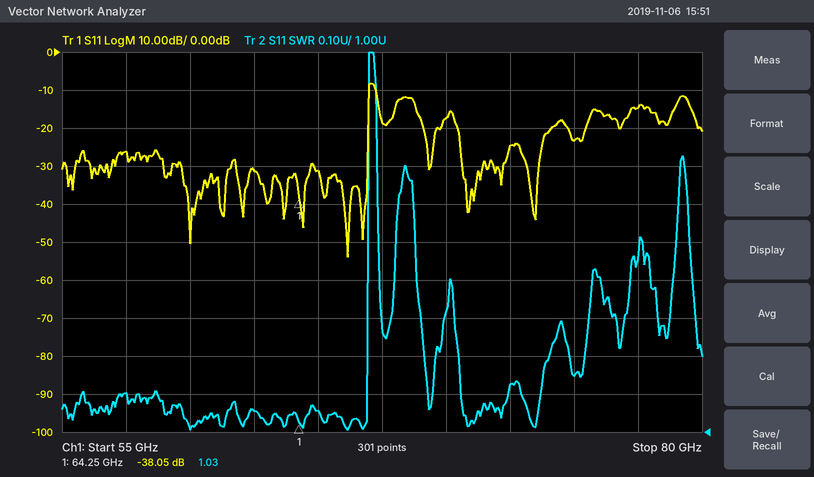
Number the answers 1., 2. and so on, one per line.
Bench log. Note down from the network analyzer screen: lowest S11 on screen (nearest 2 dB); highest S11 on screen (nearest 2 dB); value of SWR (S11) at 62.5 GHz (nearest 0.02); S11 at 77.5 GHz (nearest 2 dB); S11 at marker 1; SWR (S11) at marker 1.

1. -54 dB
2. -8 dB
3. 1.06
4. -14 dB
5. -38.05 dB
6. 1.03
